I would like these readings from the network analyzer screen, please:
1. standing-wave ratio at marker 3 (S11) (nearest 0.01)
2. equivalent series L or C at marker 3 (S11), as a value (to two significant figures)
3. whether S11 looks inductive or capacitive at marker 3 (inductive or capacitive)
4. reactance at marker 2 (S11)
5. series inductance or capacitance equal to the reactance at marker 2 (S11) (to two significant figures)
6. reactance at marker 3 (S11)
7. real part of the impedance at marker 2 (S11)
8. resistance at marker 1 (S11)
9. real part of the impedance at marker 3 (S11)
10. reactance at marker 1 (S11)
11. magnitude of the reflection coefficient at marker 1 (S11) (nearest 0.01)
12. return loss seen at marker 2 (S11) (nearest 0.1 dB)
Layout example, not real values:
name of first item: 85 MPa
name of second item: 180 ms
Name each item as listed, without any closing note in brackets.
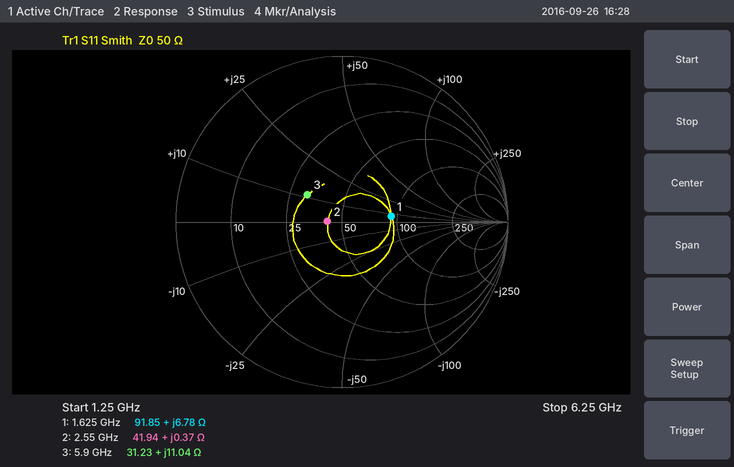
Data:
standing-wave ratio at marker 3 (S11): 1.72
equivalent series L or C at marker 3 (S11), as a value: 300 pH
whether S11 looks inductive or capacitive at marker 3: inductive
reactance at marker 2: +0.37 Ω
series inductance or capacitance equal to the reactance at marker 2 (S11): 23 pH
reactance at marker 3: +11.04 Ω
real part of the impedance at marker 2: 41.94 Ω
resistance at marker 1: 91.85 Ω
real part of the impedance at marker 3: 31.23 Ω
reactance at marker 1: +6.78 Ω
magnitude of the reflection coefficient at marker 1 (S11): 0.30
return loss seen at marker 2 (S11): 21.1 dB
